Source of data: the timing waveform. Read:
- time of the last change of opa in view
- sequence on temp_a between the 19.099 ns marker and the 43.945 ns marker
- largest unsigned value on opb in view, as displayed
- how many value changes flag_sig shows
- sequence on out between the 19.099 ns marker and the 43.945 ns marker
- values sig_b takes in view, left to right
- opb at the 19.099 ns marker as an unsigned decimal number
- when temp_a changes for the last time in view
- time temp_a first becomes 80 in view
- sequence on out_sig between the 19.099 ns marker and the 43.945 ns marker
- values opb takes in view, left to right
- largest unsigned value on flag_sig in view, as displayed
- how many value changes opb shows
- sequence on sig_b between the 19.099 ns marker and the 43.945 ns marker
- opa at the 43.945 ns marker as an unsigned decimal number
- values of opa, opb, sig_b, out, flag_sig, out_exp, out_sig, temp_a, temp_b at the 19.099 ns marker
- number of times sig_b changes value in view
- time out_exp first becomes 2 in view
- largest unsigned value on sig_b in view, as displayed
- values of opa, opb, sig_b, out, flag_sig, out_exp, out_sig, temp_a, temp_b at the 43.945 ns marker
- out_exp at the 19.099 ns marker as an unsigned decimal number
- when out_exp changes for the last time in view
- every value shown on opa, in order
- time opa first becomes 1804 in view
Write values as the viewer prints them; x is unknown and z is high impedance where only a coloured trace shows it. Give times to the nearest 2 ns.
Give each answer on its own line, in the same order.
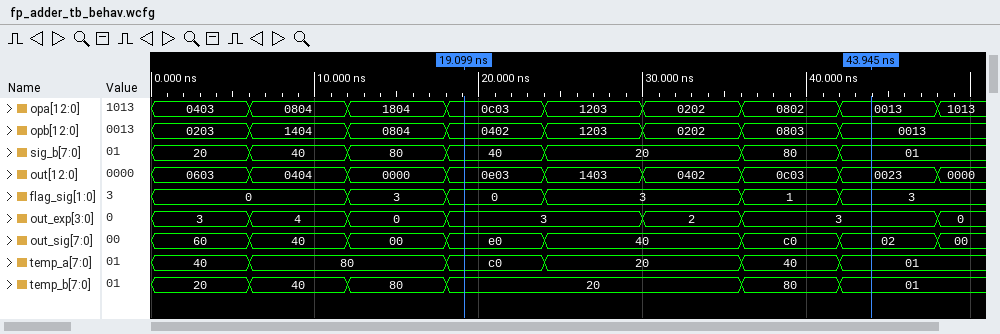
48 ns
c0, 20, 40, 01
1404
5
0e03, 1403, 0402, 0c03, 0023
20, 40, 80, 40, 20, 80, 01
1026
42 ns
6 ns
e0, 40, c0, 02
0203, 1404, 0804, 0402, 1203, 0202, 0803, 0013
3
7
40, 20, 80, 01
19
opa=0c03, opb=0402, sig_b=40, out=0e03, flag_sig=0, out_exp=3, out_sig=e0, temp_a=c0, temp_b=20
6
30 ns
80
opa=0013, opb=0013, sig_b=01, out=0023, flag_sig=3, out_exp=3, out_sig=02, temp_a=01, temp_b=01
3
48 ns
0403, 0804, 1804, 0c03, 1203, 0202, 0802, 0013, 1013
12 ns
